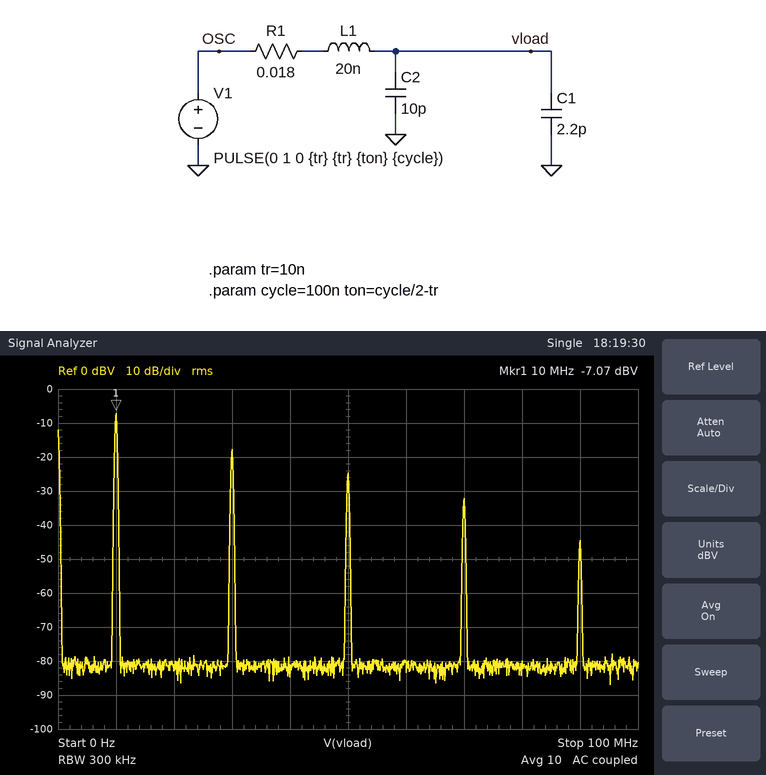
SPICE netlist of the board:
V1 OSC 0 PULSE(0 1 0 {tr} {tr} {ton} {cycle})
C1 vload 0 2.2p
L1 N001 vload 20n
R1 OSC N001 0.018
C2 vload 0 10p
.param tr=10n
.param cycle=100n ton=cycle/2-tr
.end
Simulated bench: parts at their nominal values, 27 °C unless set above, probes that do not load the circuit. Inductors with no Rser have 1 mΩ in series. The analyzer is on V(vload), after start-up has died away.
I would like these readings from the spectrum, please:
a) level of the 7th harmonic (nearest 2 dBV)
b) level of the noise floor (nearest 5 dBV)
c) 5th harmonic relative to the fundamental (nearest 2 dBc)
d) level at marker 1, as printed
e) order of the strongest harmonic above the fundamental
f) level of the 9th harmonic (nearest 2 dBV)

-32 dBV
-80 dBV
-18 dBc
-7.07 dBV
3
-44 dBV
